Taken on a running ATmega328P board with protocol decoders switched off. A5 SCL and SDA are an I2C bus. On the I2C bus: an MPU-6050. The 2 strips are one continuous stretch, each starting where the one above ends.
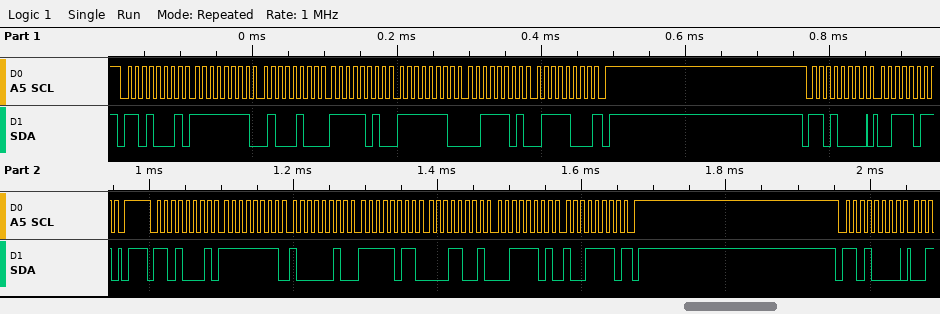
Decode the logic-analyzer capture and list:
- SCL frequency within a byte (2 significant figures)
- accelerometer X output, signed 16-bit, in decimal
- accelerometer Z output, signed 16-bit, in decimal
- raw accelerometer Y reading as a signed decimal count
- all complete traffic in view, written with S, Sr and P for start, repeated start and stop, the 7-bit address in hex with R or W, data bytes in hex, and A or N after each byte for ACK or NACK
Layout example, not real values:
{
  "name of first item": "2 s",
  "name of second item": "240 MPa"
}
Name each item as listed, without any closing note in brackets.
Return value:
{
  "SCL frequency within a byte": "100 kHz",
  "accelerometer X output, signed 16-bit, in decimal": "-126",
  "accelerometer Z output, signed 16-bit, in decimal": "15774",
  "raw accelerometer Y reading as a signed decimal count": "-1255",
  "all complete traffic in view, written with S, Sr and P for start, repeated start and stop, the 7-bit address in hex with R or W, data bytes in hex, and A or N after each byte for ACK or NACK": "S 68R A FF A 44 A FA A FE A 3D A 78 N P S 68W A 3B A P S 68R A FF A 82 A FB A 19 A 3D A 9E N P S 68W A"
}
